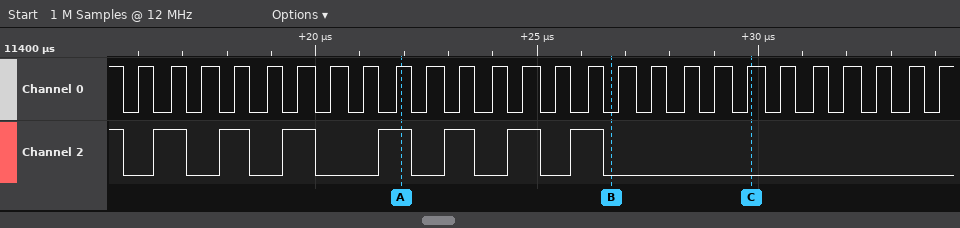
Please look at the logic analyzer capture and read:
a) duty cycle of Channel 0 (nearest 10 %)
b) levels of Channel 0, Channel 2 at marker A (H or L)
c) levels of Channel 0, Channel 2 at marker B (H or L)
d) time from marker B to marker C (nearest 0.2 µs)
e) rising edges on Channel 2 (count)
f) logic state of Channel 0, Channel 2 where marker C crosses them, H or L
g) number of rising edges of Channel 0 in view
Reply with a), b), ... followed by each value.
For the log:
a) 50 %
b) Channel 0=H, Channel 2=H
c) Channel 0=L, Channel 2=L
d) 3.2 µs
e) 7
f) Channel 0=H, Channel 2=L
g) 26
